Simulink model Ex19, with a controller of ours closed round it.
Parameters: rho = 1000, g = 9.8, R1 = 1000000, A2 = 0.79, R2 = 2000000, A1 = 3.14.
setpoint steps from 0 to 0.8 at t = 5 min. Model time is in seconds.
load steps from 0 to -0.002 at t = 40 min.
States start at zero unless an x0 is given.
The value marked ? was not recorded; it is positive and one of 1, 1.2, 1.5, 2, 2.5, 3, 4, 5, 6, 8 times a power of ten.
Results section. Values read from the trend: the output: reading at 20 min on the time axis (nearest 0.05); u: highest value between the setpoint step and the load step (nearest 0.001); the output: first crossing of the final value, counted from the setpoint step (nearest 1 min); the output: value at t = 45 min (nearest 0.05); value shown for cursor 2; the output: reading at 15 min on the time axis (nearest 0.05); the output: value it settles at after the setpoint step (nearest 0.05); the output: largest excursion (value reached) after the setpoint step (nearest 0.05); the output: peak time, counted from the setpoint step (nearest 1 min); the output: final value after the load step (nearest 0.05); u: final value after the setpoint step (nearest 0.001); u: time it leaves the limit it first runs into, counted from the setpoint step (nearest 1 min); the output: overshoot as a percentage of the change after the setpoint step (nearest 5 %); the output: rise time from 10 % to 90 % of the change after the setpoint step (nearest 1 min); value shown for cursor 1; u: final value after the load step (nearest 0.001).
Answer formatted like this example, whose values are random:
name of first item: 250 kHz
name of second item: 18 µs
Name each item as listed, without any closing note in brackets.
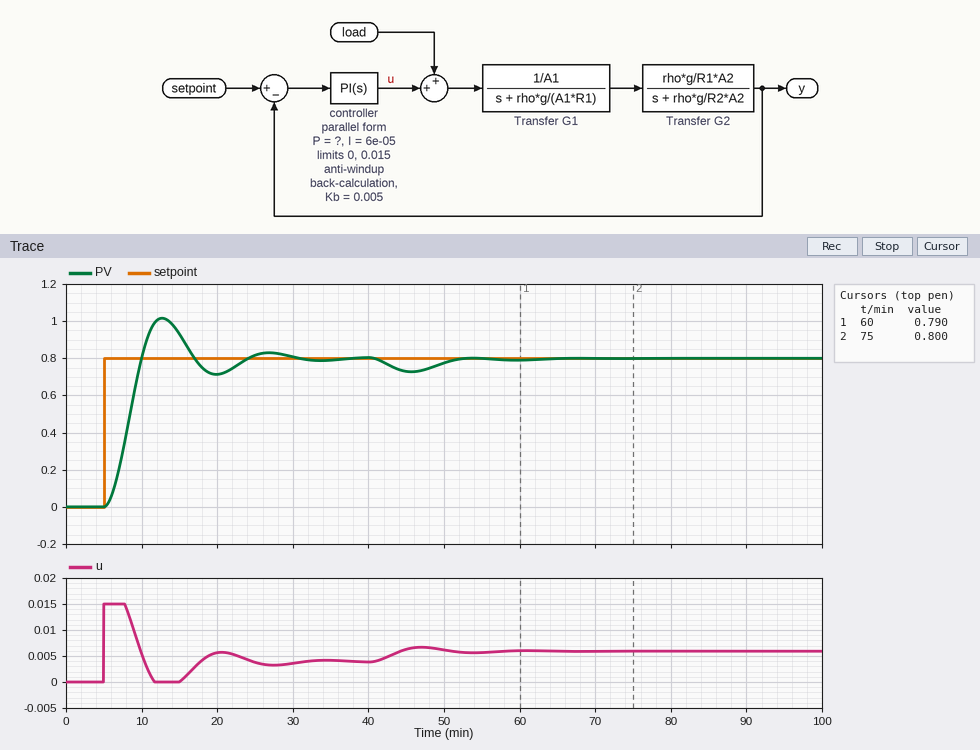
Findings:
the output: reading at 20 min on the time axis: 0.70
u: highest value between the setpoint step and the load step: 0.015
the output: first crossing of the final value, counted from the setpoint step: 5 min
the output: value at t = 45 min: 0.75
value shown for cursor 2: 0.800
the output: reading at 15 min on the time axis: 0.95
the output: value it settles at after the setpoint step: 0.80
the output: largest excursion (value reached) after the setpoint step: 1.00
the output: peak time, counted from the setpoint step: 8 min
the output: final value after the load step: 0.80
u: final value after the setpoint step: 0.004
u: time it leaves the limit it first runs into, counted from the setpoint step: 3 min
the output: overshoot as a percentage of the change after the setpoint step: 25 %
the output: rise time from 10 % to 90 % of the change after the setpoint step: 3 min
value shown for cursor 1: 0.790
u: final value after the load step: 0.006
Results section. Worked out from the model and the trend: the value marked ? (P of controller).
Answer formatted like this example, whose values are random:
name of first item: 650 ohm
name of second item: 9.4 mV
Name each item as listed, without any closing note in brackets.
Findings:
the value marked ?: 0.025
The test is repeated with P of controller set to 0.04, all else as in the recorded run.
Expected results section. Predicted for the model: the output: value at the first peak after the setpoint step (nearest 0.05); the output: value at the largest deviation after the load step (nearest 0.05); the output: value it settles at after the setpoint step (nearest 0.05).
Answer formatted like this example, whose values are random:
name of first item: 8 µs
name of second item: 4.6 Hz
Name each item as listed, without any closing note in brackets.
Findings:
the output: value at the first peak after the setpoint step: 0.90
the output: value at the largest deviation after the load step: 0.75
the output: value it settles at after the setpoint step: 0.80
